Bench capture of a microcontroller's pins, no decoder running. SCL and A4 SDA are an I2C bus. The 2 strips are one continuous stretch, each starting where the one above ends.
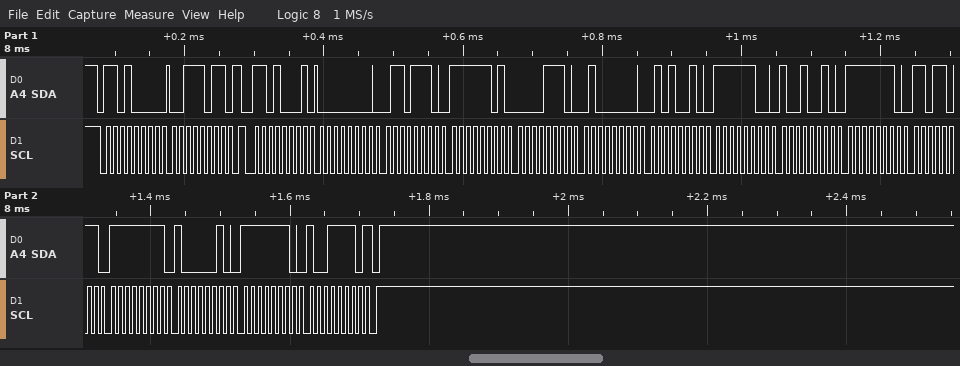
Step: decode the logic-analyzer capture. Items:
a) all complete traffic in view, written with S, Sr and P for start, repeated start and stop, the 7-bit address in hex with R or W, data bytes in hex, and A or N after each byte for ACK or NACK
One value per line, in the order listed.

S 68W A 3B A Sr 68R A 00 A 6E A FD A 0E A 40 A 52 A FC A 92 A FE A DB A FF A 82 A FE A 9E N P
